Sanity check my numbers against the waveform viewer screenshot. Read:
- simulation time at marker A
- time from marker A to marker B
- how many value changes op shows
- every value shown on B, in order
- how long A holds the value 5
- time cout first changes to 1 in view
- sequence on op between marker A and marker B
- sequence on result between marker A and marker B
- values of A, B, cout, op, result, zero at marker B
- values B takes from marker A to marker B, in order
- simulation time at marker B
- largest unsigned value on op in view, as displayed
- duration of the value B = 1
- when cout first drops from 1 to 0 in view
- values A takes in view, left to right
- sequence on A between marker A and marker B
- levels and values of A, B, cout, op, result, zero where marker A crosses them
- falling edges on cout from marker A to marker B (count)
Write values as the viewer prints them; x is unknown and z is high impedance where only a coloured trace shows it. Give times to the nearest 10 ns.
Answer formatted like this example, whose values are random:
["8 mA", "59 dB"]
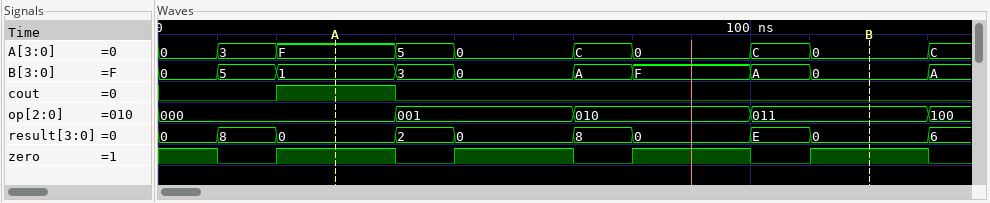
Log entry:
["30 ns", "90 ns", "4", "0, 5, 1, 3, 0, A, F, A, 0, A", "10 ns", "20 ns", "000, 001, 010, 011", "0, 2, 0, 8, 0, E, 0", "A=0, B=0, cout=0, op=011, result=0, zero=1", "1, 3, 0, A, F, A, 0", "120 ns", "100", "20 ns", "40 ns", "0, 3, F, 5, 0, C, 0, C, 0, C", "F, 5, 0, C, 0, C, 0", "A=F, B=1, cout=1, op=000, result=0, zero=1", "1"]
